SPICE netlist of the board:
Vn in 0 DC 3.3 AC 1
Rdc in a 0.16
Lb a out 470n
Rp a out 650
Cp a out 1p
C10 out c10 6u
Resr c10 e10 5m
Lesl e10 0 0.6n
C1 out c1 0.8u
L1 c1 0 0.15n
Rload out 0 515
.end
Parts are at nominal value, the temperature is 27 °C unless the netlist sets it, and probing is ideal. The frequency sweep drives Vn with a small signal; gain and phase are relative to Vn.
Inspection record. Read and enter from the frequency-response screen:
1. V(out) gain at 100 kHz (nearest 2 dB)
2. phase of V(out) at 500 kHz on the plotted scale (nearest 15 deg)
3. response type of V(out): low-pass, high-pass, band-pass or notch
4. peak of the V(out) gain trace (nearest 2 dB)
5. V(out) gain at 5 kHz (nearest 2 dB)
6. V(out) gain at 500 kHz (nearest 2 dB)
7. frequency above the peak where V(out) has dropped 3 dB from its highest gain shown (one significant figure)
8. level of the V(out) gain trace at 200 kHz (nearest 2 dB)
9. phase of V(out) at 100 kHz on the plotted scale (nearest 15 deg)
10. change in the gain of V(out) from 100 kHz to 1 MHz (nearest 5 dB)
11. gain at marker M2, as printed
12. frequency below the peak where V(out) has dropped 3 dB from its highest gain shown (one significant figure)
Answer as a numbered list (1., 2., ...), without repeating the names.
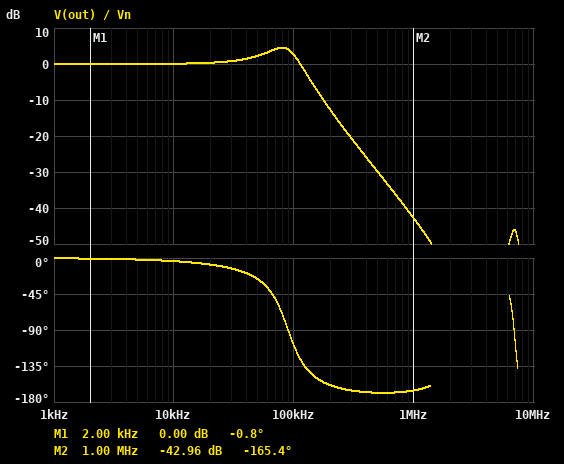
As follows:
1. 2 dB
2. -165 deg
3. low-pass
4. 4 dB
5. 0 dB
6. -30 dB
7. 100 kHz
8. -12 dB
9. -105 deg
10. -45 dB
11. -42.96 dB
12. 40 kHz
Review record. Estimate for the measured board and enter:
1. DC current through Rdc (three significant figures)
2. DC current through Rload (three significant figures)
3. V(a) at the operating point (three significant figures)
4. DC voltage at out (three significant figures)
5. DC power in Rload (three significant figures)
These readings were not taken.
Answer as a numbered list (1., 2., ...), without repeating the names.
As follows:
1. 6.41 mA
2. 6.41 mA
3. 3.30 V
4. 3.30 V
5. 21.1 mW
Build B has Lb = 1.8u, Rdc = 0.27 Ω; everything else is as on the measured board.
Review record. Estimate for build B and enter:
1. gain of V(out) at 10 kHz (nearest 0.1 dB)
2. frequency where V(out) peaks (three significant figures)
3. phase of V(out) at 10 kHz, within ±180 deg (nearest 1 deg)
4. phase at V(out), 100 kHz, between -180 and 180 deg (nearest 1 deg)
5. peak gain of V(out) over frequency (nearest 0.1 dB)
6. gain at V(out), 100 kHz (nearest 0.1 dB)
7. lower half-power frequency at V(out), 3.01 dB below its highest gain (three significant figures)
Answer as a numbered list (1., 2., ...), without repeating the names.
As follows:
1. 0.4 dB
2. 42.1 kHz
3. -7 deg
4. -162 deg
5. 5.8 dB
6. -12.1 dB
7. 26.6 kHz
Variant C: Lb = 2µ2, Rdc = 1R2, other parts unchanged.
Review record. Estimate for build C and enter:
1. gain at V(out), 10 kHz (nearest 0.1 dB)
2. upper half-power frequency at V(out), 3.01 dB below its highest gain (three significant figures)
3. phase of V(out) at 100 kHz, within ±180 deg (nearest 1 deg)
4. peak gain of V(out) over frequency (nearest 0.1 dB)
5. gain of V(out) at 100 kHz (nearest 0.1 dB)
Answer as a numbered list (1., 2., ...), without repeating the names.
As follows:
1. -0.6 dB
2. 24.5 kHz
3. -133 deg
4. 0 dB
5. -17.1 dB
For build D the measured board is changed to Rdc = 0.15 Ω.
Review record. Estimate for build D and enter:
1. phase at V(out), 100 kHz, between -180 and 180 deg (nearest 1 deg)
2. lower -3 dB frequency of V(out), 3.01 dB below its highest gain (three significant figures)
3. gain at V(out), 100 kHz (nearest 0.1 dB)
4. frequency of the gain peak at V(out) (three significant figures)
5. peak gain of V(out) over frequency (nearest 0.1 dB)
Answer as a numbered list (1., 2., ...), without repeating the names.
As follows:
1. -111 deg
2. 46.0 kHz
3. 3.0 dB
4. 81.0 kHz
5. 5.0 dB
